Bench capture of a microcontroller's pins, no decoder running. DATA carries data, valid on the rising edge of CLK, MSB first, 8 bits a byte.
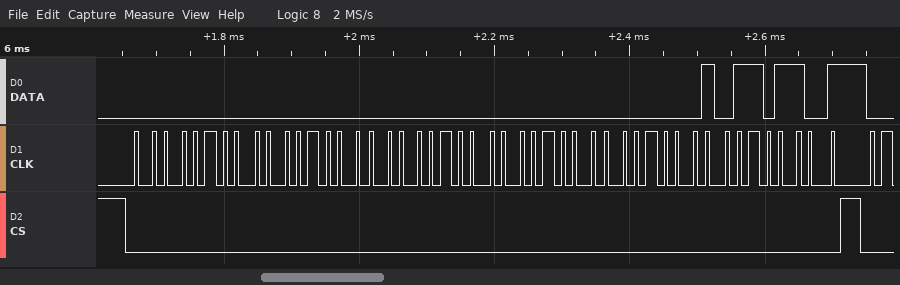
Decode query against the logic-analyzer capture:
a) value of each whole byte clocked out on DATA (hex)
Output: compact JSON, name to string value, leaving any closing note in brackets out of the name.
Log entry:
{"value of each whole byte clocked out on DATA": "0x00 0x00 0x00 0x00 0x01 0x6D"}
